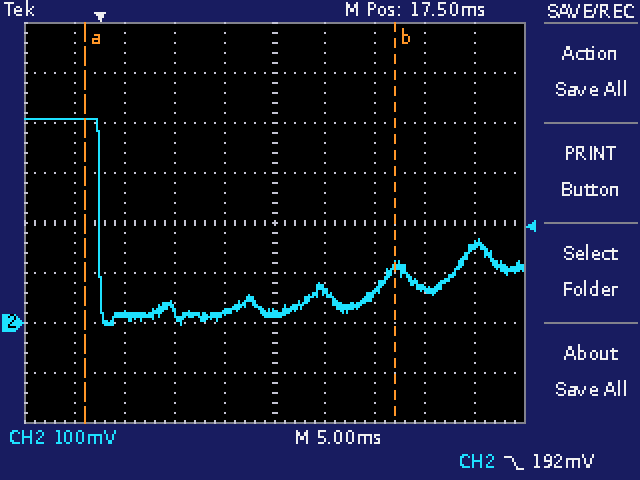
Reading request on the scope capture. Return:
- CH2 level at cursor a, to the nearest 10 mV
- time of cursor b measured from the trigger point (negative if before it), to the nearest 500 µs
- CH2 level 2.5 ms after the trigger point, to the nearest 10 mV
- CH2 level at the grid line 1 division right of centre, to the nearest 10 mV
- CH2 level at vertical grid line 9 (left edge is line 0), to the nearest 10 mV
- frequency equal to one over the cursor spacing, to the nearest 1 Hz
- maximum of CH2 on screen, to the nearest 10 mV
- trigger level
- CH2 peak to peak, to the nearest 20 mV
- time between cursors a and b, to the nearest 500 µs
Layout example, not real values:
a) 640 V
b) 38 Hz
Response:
a) 410 mV
b) +29.5 ms
c) 20 mV
d) 60 mV
e) 150 mV
f) 32 Hz
g) 410 mV
h) 192 mV
i) 420 mV
j) 31.0 ms
